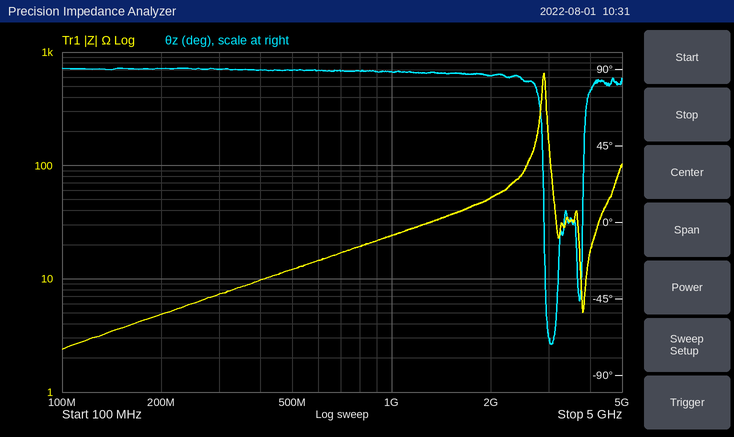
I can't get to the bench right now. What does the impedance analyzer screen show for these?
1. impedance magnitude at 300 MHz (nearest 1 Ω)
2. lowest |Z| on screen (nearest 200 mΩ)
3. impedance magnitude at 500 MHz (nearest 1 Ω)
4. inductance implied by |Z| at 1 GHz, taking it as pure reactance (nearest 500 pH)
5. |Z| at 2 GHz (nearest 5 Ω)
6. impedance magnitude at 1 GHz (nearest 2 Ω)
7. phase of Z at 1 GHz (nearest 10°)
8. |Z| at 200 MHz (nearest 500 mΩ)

7 Ω
2.4 Ω
12 Ω
4.0 nH
50 Ω
24 Ω
90°
5.0 Ω
